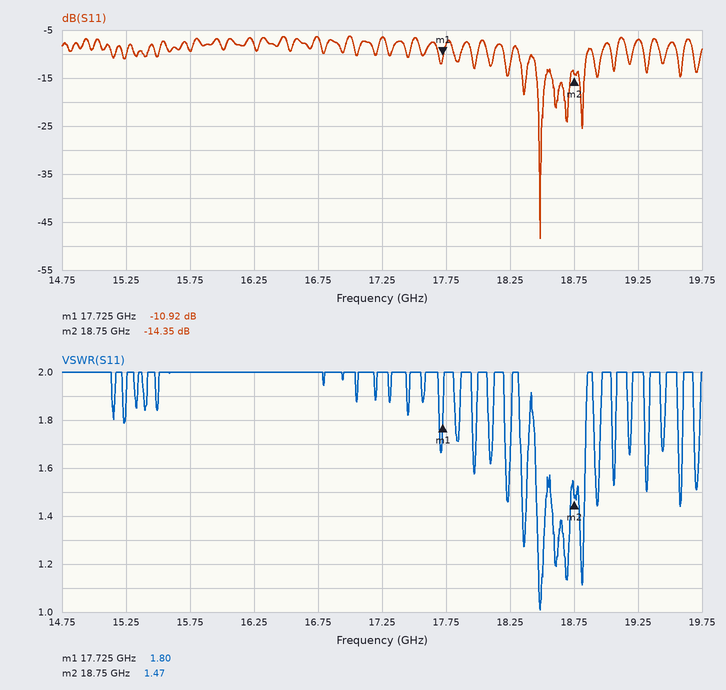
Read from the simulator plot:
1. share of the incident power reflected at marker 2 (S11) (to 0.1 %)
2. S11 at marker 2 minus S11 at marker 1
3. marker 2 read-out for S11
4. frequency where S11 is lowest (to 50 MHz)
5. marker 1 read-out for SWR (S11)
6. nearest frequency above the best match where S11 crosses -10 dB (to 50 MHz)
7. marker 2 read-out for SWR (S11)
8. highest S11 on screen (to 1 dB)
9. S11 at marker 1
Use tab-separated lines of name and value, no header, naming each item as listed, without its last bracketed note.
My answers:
share of the incident power reflected at marker 2 (S11)	3.7 %
S11 at marker 2 minus S11 at marker 1	-3.43 dB
marker 2 read-out for S11	-14.35 dB
frequency where S11 is lowest	18.50 GHz
marker 1 read-out for SWR	1.80
nearest frequency above the best match where S11 crosses -10 dB	18.85 GHz
marker 2 read-out for SWR	1.47
highest S11 on screen	-6 dB
S11 at marker 1	-10.92 dB
